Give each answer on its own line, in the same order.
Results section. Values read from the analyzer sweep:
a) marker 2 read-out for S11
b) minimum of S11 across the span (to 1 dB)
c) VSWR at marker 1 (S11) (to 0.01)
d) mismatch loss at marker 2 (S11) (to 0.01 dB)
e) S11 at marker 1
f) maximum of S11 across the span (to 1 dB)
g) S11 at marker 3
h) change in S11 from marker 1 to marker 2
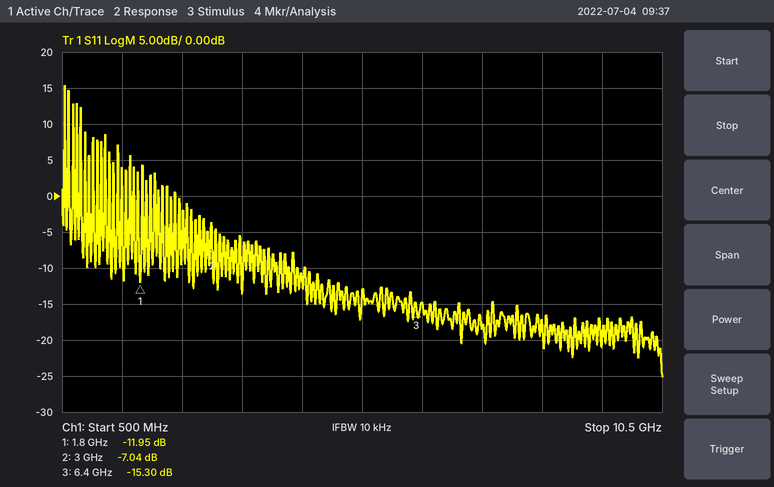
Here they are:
-7.04 dB
-25 dB
1.68
0.96 dB
-11.95 dB
15 dB
-15.30 dB
4.91 dB
